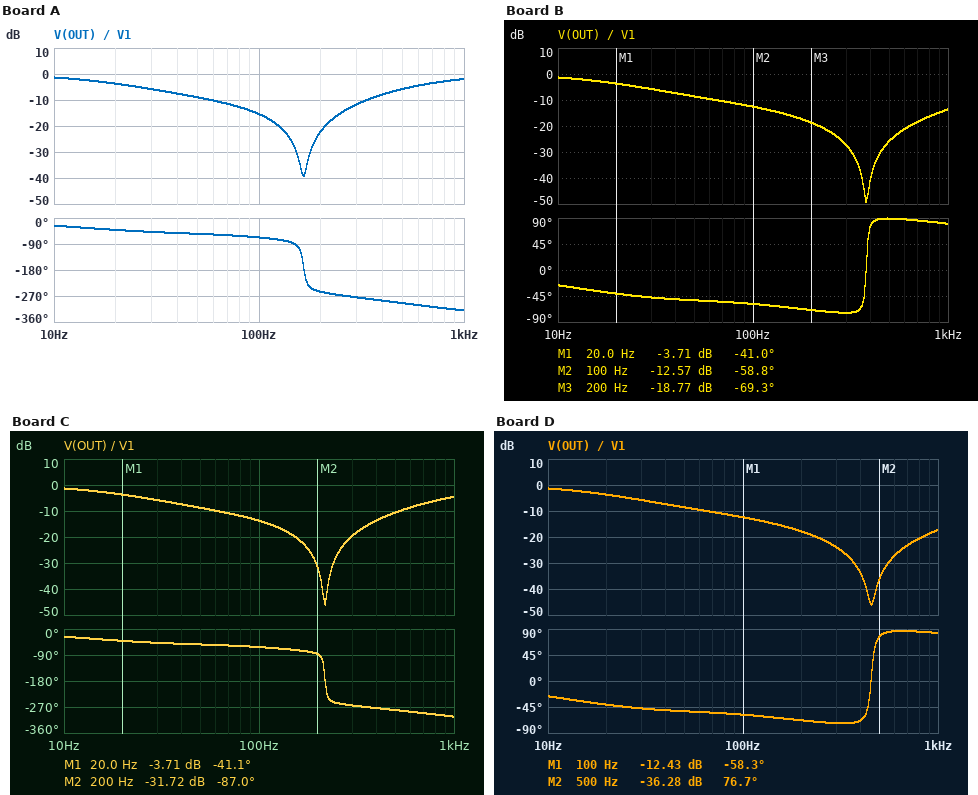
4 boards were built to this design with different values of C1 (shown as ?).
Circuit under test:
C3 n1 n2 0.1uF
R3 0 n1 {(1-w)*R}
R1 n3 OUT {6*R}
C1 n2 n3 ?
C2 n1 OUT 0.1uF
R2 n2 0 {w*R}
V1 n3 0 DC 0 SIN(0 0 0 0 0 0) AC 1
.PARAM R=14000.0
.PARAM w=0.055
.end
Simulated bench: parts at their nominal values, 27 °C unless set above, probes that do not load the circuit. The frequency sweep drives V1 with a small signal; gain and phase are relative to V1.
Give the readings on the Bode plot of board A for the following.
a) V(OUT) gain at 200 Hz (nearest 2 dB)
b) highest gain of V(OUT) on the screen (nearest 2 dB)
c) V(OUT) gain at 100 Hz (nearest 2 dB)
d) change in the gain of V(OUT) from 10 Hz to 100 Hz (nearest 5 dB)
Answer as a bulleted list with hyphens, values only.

- -22 dB
- -2 dB
- -16 dB
- -15 dB
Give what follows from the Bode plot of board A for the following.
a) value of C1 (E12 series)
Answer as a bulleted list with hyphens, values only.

- 330 nF
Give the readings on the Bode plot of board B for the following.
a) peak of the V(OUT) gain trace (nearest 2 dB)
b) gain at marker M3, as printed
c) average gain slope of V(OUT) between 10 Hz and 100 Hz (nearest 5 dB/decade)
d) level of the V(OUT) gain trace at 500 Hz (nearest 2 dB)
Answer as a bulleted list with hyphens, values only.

- -2 dB
- -18.77 dB
- -10 dB/decade
- -26 dB
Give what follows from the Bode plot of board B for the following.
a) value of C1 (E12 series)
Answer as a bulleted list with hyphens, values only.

- 56 nF
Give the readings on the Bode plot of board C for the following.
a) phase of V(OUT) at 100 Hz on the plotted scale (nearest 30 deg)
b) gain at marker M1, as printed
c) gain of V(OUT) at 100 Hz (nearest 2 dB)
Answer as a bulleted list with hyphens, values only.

- -60 deg
- -3.71 dB
- -14 dB
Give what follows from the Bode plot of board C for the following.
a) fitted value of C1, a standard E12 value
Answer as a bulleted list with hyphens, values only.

- 180 nF
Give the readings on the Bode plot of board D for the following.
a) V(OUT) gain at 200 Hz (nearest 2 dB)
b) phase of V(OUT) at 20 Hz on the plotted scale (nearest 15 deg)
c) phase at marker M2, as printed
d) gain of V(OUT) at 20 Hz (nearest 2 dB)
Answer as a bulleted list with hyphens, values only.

- -18 dB
- -45 deg
- 76.7 deg
- -4 dB
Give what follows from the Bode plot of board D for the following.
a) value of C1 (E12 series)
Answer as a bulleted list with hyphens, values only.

- 39 nF
